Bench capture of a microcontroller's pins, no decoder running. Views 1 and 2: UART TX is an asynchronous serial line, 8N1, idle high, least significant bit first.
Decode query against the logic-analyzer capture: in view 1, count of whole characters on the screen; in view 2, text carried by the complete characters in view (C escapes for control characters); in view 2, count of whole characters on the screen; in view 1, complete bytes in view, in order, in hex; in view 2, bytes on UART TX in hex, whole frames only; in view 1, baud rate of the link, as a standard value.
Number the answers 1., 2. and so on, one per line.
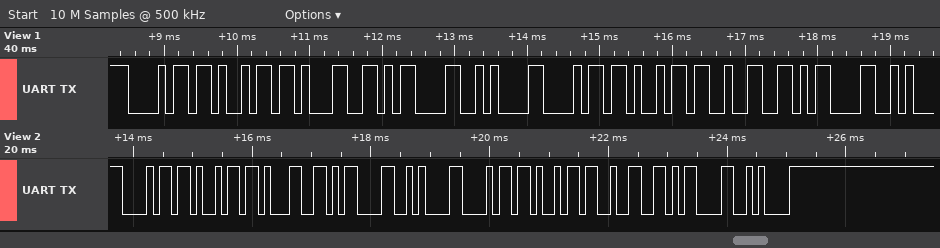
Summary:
1. 9
2. "hi1\r\nhi2\r\n"
3. 10
4. 68 69 31 0D 0A 68 69 32 0D
5. 0x68 0x69 0x31 0x0D 0x0A 0x68 0x69 0x32 0x0D 0x0A
6. 9600 baud
